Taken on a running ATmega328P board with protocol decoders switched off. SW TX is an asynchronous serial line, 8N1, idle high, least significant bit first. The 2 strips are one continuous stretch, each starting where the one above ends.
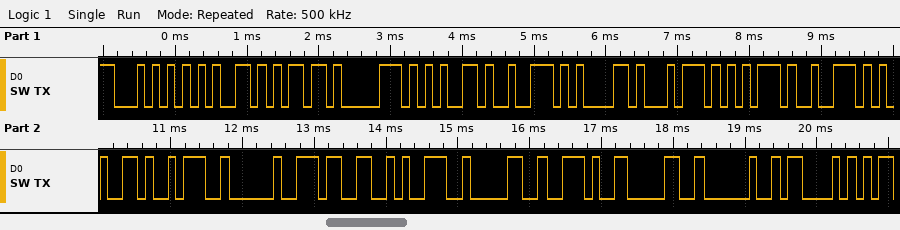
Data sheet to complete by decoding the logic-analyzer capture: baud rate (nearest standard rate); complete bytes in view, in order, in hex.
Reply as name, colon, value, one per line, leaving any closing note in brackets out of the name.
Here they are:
baud rate: 9600 baud
complete bytes in view, in order, in hex: 54 65 6D 70 65 72 61 74 75 72 65 3A 20 33 39 30 2E 30 20 43
